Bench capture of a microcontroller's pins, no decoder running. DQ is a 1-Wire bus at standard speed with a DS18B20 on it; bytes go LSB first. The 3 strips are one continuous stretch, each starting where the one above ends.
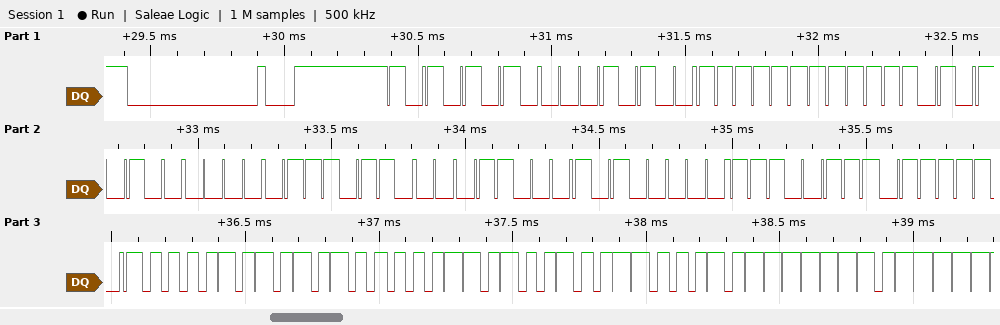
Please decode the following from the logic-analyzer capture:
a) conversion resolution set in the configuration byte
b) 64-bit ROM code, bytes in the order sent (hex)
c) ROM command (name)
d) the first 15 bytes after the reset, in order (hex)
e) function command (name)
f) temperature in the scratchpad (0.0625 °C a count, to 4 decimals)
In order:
12 bits
28 FF AF 02 6E 18 05 E7
Match ROM
55 28 FF AF 02 6E 18 05 E7 BE 50 05 4B 46 7F
Read Scratchpad
85.0000 °C
